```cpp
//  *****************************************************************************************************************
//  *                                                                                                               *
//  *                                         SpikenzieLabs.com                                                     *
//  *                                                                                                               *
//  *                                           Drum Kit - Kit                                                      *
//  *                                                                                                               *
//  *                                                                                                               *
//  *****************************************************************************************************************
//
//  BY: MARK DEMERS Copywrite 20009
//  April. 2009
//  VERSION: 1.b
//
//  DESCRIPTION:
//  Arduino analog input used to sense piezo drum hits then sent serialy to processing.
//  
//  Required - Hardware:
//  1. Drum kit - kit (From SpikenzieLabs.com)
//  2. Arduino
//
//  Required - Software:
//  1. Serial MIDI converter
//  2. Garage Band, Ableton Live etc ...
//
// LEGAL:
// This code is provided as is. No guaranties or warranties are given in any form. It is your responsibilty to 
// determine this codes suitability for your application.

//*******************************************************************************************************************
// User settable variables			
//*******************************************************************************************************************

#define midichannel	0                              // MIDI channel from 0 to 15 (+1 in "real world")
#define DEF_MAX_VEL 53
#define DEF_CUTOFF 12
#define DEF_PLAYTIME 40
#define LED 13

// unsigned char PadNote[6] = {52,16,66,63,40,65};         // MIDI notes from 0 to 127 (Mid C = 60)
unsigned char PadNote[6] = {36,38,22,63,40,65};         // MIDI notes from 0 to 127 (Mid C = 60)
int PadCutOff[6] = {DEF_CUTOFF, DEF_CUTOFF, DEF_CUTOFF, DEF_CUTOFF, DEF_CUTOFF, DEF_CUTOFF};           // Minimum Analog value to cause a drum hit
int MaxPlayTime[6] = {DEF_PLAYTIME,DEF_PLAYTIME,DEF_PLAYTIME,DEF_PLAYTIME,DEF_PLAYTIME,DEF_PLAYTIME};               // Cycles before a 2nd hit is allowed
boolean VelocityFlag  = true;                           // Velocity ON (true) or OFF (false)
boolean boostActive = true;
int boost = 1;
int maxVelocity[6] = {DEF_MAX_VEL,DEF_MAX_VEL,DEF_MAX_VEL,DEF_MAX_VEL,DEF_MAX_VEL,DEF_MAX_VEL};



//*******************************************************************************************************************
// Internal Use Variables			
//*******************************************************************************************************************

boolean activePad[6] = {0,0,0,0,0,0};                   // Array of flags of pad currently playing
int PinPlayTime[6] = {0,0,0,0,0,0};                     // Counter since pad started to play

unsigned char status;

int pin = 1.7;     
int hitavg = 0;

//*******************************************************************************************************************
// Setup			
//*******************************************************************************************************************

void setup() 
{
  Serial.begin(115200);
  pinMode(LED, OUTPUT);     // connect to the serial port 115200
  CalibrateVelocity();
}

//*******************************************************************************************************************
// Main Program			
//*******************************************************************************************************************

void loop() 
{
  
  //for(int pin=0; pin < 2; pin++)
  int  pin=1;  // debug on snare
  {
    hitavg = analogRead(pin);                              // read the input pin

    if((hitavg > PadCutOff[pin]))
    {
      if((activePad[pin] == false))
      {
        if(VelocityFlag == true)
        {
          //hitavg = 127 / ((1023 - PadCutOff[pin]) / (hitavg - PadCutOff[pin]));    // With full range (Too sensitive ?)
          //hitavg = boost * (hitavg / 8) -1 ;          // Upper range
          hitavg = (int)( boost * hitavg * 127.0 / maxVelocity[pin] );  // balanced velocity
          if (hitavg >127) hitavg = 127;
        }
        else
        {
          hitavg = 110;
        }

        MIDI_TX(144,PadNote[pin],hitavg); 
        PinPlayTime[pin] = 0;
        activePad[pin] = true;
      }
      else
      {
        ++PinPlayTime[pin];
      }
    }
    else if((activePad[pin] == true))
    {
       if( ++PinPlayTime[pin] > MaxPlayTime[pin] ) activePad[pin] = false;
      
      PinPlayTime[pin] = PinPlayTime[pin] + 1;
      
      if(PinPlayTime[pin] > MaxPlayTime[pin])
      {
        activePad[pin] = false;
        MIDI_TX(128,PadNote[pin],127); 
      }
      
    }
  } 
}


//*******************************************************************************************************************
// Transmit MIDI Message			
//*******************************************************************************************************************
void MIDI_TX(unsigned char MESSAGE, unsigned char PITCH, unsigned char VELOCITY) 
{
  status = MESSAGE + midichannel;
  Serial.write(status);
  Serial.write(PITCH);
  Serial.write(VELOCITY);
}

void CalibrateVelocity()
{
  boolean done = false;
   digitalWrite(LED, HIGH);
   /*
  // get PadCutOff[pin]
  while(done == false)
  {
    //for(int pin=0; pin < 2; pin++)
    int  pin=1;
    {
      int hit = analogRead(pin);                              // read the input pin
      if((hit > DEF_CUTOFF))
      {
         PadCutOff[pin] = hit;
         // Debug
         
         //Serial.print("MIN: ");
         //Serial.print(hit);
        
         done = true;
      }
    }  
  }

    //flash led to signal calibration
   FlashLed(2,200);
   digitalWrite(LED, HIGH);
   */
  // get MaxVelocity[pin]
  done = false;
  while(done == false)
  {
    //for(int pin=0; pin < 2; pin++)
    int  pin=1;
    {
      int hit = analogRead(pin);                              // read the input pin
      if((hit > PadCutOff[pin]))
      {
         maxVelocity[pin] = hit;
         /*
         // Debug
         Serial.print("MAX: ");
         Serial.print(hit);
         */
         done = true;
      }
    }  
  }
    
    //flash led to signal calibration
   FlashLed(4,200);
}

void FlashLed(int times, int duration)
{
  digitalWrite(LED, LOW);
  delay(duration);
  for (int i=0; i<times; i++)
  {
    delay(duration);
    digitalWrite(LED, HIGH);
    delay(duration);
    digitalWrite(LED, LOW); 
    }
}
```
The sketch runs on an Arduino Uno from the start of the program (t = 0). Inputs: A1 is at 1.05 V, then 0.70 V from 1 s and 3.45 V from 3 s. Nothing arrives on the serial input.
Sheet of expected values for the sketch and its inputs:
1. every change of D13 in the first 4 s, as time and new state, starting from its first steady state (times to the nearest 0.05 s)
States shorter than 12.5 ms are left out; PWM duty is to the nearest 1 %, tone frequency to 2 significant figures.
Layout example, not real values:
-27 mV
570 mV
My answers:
0 s low; 0.4 s high; 0.6 s low; 0.8 s high; 1 s low; 1.2 s high; 1.4 s low; 1.6 s high; 1.8 s low
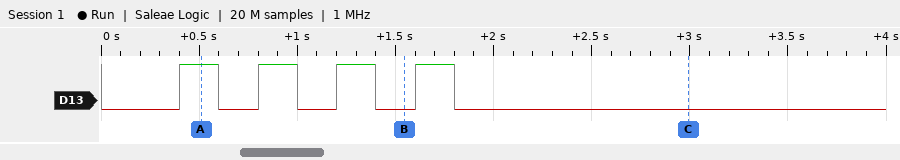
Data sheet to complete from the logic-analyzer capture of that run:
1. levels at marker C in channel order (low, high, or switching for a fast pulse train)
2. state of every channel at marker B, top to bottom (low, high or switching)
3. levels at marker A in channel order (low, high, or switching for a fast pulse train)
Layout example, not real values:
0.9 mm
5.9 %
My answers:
D13 low
D13 low
D13 high
